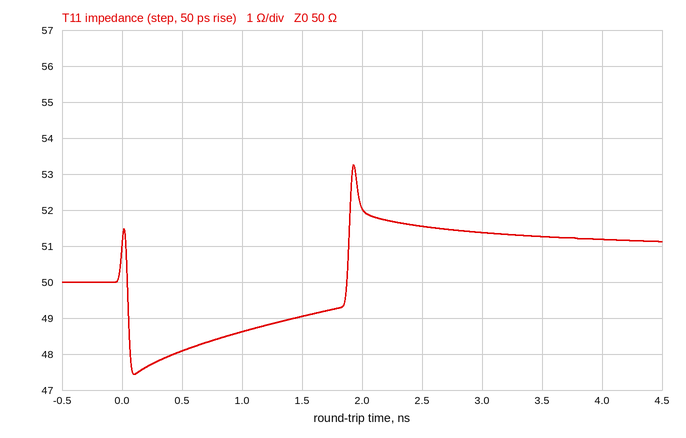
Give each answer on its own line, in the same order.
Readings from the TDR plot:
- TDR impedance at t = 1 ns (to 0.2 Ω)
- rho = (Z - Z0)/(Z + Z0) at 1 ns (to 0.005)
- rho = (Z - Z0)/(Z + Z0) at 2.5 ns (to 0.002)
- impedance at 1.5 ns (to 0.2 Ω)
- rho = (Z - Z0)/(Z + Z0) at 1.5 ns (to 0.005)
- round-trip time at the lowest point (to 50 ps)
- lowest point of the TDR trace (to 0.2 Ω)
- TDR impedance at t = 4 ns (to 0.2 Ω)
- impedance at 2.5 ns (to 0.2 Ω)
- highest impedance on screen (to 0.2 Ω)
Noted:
48.6 Ω
-0.015
+0.016
49.0 Ω
-0.010
100 ps
47.4 Ω
51.2 Ω
51.6 Ω
53.2 Ω
